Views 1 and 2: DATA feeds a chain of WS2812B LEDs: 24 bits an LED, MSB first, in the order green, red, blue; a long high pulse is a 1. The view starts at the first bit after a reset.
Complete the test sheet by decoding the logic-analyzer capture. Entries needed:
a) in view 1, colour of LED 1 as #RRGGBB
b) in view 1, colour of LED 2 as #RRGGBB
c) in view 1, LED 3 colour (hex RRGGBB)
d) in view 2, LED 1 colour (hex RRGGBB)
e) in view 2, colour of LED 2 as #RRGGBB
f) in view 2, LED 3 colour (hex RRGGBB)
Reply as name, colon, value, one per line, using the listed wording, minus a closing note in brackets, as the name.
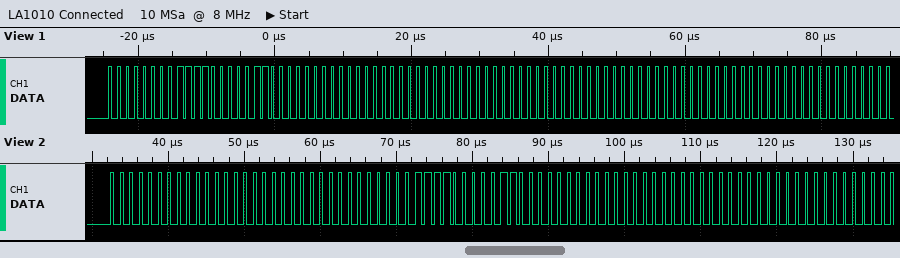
in view 1, colour of LED 1 as #RRGGBB: #F00060
in view 1, colour of LED 2 as #RRGGBB: #000000
in view 1, LED 3 colour: #000000
in view 2, LED 1 colour: #000000
in view 2, colour of LED 2 as #RRGGBB: #F00060
in view 2, LED 3 colour: #000000
